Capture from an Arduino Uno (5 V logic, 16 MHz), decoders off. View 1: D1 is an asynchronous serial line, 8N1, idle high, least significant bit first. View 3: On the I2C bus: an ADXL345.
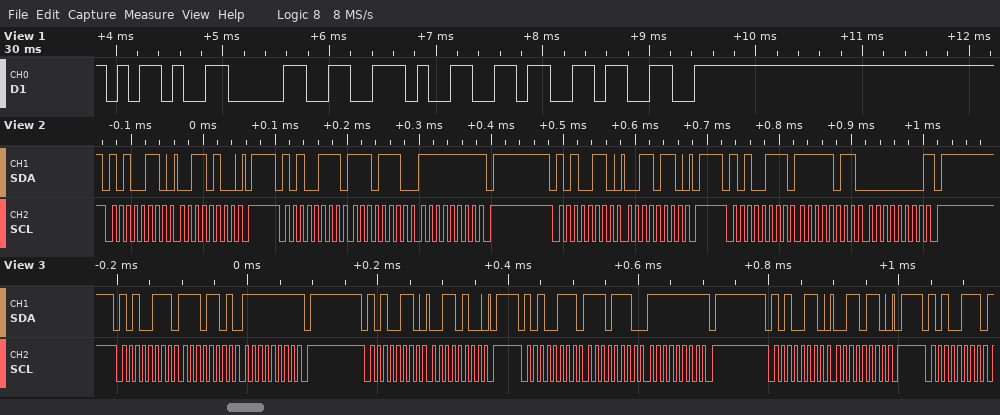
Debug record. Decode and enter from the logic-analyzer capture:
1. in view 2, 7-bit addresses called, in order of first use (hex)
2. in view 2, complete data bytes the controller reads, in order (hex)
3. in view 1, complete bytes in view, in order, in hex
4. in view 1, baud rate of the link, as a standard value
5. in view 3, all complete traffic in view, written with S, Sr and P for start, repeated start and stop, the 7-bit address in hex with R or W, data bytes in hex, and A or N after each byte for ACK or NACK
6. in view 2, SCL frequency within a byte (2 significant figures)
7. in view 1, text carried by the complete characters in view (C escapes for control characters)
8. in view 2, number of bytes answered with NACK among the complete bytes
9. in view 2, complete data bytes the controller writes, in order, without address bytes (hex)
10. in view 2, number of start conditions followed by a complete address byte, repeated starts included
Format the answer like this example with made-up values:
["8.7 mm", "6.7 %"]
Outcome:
["0x53", "EE FF FB 00", "2D 30 2E 36 33", "9600 baud", "S 53R A ED A FF N P S 53W A 34 A P S 53R A EE A FF N P S 53W A 36 A P S 53R A", "100 kHz", "\"-0.63\"", "2", "34 36", "4"]
